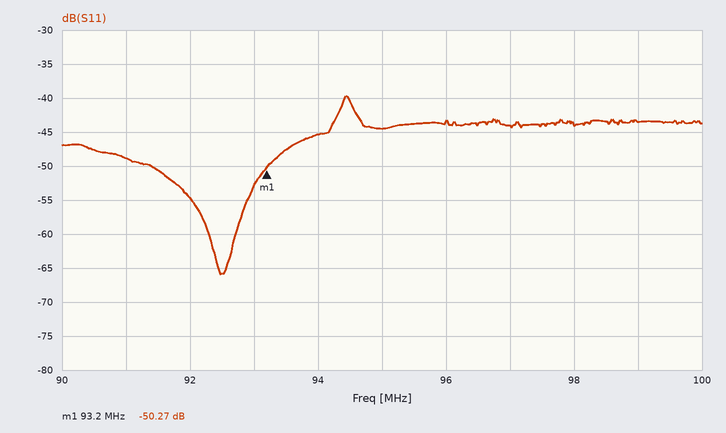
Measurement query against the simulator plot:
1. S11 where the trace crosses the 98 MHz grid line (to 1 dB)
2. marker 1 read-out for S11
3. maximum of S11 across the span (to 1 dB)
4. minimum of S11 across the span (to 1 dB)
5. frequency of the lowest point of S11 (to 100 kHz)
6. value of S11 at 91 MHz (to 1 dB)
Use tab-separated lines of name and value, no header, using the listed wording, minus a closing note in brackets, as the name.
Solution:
S11 where the trace crosses the 98 MHz grid line	-44 dB
marker 1 read-out for S11	-50.27 dB
maximum of S11 across the span	-40 dB
minimum of S11 across the span	-66 dB
frequency of the lowest point of S11	92.5 MHz
value of S11 at 91 MHz	-49 dB
